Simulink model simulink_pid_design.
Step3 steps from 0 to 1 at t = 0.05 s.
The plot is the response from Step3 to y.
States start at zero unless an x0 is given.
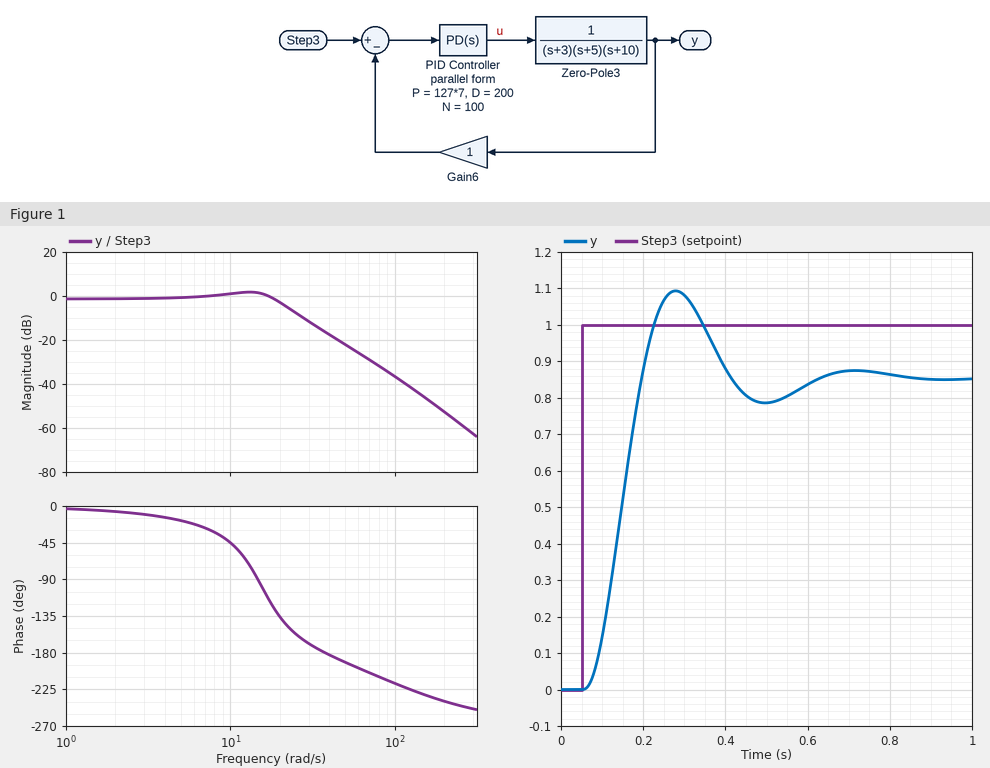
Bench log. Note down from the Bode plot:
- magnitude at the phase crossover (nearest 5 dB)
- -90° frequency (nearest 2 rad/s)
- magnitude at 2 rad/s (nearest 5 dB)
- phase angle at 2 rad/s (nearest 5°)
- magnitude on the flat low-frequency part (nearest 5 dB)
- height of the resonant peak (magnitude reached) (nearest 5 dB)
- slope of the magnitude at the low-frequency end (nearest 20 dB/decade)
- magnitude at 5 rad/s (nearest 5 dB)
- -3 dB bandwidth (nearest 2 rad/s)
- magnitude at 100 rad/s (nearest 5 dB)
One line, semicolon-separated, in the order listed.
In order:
-15 dB; 14 rad/s; 0 dB; -5°; 0 dB; 0 dB; 0 dB/decade; 0 dB; 22 rad/s; -35 dB
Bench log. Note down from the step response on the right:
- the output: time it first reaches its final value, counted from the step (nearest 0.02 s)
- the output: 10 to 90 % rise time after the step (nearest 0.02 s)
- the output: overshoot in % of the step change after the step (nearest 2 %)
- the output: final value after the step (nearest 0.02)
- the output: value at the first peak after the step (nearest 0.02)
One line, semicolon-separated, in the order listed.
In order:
0.14 s; 0.10 s; 28 %; 0.86; 1.10
